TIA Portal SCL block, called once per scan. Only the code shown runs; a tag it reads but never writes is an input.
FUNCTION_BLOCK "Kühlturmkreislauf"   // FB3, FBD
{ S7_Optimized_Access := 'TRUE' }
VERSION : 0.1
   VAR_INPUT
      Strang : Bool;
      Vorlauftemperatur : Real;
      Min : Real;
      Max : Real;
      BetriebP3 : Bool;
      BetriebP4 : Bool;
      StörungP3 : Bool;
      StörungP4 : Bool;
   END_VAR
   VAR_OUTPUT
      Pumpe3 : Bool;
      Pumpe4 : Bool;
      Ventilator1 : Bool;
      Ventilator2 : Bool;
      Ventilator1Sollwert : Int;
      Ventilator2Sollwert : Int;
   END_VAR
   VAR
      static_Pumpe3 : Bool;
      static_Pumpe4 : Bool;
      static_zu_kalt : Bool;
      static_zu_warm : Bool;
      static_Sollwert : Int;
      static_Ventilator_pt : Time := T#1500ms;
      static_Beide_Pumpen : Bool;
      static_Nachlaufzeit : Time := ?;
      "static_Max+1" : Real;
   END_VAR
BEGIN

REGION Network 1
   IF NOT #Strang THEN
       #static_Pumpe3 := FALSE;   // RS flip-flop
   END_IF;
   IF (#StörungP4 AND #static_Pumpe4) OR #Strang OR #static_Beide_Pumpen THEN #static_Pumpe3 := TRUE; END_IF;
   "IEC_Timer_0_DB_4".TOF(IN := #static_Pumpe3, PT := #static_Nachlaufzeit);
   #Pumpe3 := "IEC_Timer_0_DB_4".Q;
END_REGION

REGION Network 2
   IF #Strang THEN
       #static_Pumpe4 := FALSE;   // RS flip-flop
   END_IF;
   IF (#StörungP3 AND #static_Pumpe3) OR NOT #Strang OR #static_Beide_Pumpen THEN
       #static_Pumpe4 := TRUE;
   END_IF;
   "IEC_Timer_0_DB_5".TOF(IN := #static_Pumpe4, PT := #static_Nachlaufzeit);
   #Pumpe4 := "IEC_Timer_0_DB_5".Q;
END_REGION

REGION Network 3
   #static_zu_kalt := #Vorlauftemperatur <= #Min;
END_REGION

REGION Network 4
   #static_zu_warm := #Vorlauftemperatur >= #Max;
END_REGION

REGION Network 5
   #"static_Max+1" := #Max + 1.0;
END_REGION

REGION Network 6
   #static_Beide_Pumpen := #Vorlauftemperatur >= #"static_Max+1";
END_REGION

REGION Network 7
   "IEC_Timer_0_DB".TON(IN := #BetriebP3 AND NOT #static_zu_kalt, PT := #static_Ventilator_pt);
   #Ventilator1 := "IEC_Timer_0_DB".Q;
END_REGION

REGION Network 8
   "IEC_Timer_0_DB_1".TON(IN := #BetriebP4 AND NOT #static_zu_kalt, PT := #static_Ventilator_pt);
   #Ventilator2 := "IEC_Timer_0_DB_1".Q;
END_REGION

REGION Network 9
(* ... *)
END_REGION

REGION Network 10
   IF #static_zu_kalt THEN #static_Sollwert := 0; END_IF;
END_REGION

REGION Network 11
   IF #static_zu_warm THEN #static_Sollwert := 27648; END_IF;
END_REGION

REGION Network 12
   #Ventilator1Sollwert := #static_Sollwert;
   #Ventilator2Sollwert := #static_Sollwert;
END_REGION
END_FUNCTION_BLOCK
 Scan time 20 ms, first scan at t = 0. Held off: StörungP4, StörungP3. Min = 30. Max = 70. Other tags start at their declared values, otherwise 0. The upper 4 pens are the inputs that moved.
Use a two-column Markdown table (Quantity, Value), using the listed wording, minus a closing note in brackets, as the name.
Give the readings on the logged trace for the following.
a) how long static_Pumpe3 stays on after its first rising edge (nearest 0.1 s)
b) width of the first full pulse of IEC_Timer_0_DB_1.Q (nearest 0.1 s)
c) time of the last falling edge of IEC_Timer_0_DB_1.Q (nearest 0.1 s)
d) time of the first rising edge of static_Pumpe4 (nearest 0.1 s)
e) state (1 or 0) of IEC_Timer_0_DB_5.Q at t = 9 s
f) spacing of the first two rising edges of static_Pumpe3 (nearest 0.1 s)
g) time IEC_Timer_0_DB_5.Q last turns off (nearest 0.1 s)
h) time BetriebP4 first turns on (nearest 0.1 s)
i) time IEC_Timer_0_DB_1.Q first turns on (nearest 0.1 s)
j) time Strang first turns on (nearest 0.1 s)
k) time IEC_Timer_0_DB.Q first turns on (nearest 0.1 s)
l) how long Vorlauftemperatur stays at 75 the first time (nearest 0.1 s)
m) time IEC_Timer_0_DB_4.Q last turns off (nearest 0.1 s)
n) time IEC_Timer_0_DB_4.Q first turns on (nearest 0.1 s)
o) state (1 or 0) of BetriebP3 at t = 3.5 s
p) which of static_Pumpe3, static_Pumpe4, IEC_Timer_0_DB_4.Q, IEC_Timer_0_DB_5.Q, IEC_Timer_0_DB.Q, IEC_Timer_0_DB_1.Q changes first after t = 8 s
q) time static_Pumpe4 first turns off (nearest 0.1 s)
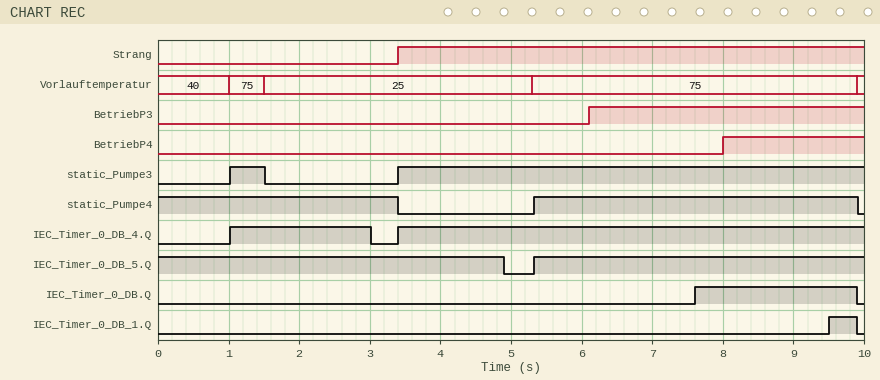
| Quantity | Value |
|---|---|
| how long static_Pumpe3 stays on after its first rising edge | 0.5 s |
| width of the first full pulse of IEC_Timer_0_DB_1.Q | 0.4 s |
| time of the last falling edge of IEC_Timer_0_DB_1.Q | 9.9 s |
| time of the first rising edge of static_Pumpe4 | 5.3 s |
| state (1 or 0) of IEC_Timer_0_DB_5.Q at t = 9 s | 1 |
| spacing of the first two rising edges of static_Pumpe3 | 2.4 s |
| time IEC_Timer_0_DB_5.Q last turns off | 4.9 s |
| time BetriebP4 first turns on | 8.0 s |
| time IEC_Timer_0_DB_1.Q first turns on | 9.5 s |
| time Strang first turns on | 3.4 s |
| time IEC_Timer_0_DB.Q first turns on | 7.6 s |
| how long Vorlauftemperatur stays at 75 the first time | 0.5 s |
| time IEC_Timer_0_DB_4.Q last turns off | 3.0 s |
| time IEC_Timer_0_DB_4.Q first turns on | 1.0 s |
| state (1 or 0) of BetriebP3 at t = 3.5 s | 0 |
| which of static_Pumpe3, static_Pumpe4, IEC_Timer_0_DB_4.Q, IEC_Timer_0_DB_5.Q, IEC_Timer_0_DB.Q, IEC_Timer_0_DB_1.Q changes first after t = 8 s | IEC_Timer_0_DB_1.Q |
| time static_Pumpe4 first turns off | 3.4 s |
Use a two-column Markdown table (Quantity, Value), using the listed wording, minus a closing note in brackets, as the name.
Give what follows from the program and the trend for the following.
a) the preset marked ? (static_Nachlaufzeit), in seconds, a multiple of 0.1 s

| Quantity | Value |
|---|---|
| the preset marked ? (static_Nachlaufzeit), in seconds, a multiple of 0.1 s | 1.5 s |
